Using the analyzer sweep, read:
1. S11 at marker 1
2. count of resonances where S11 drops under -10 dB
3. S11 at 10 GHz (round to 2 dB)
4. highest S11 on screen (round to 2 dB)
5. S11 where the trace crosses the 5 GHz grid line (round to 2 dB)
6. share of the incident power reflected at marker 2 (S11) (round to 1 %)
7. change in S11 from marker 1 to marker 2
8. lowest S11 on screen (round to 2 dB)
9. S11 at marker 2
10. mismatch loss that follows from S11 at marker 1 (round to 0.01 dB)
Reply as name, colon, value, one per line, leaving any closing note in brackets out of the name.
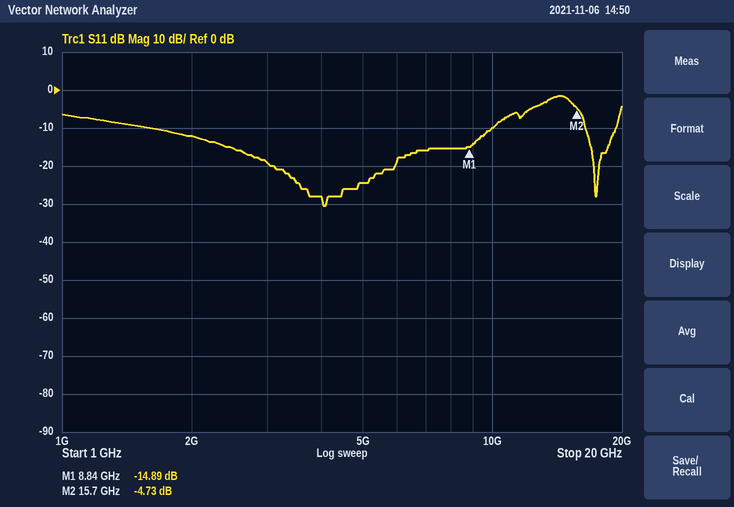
S11 at marker 1: -14.89 dB
count of resonances where S11 drops under -10 dB: 2
S11 at 10 GHz: -10 dB
highest S11 on screen: -2 dB
S11 where the trace crosses the 5 GHz grid line: -24 dB
share of the incident power reflected at marker 2 (S11): 34 %
change in S11 from marker 1 to marker 2: 10.16 dB
lowest S11 on screen: -30 dB
S11 at marker 2: -4.73 dB
mismatch loss that follows from S11 at marker 1: 0.14 dB
